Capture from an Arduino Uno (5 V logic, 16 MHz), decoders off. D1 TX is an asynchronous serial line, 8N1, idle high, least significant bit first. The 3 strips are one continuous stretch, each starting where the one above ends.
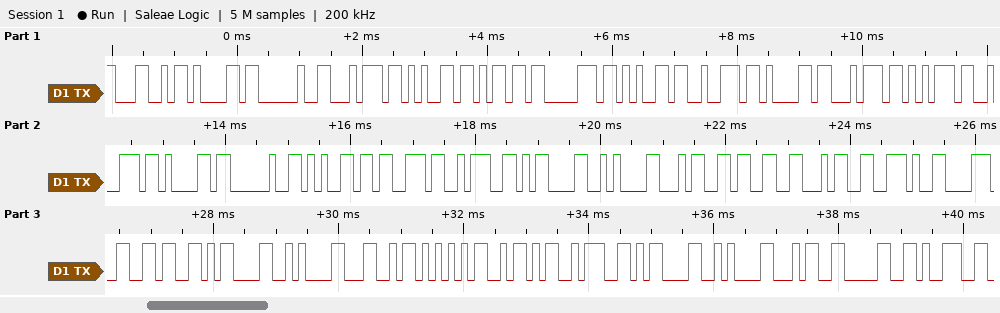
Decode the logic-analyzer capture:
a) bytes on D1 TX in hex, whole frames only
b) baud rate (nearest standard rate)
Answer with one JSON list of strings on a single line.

["4C 61 20 74 65 6D 70 65 72 61 74 75 72 61 20 65 73 3A 0D 0A 34 33 34 2E 38 36 0D 0A 4C 55 5A 3A 0D 0A 34 30 39", "9600 baud"]
